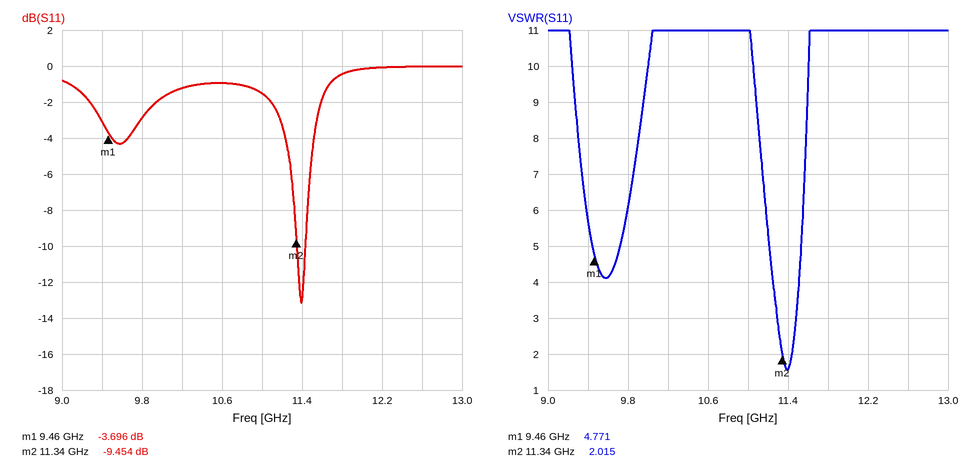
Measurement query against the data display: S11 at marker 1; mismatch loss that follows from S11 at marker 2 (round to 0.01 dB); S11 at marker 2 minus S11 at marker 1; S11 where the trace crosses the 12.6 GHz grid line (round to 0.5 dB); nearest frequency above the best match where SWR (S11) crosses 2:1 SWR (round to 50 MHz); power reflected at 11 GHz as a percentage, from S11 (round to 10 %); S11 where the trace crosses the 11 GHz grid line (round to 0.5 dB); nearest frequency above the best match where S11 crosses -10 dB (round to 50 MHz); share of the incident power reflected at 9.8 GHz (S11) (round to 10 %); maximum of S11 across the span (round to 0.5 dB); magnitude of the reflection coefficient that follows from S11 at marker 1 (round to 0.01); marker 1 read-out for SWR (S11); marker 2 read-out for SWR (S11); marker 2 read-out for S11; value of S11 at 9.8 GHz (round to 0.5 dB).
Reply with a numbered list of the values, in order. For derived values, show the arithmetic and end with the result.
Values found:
1. -3.696 dB
2. −10 log10(1 − 10^(-9.454/10)) ≈ 0.52 dB
3. -9.454 − (-3.696) = -5.758 dB
4. 0.0 dB
5. 11.45 GHz
6. 10^(-1.5/10) ≈ 70.8 %, so 70 % to the nearest 10 %
7. -1.5 dB
8. 11.45 GHz
9. 10^(-3/10) ≈ 50 %
10. 0.0 dB
11. 10^(-3.696/20) ≈ 0.65
12. 4.771
13. 2.015
14. -9.454 dB
15. -3.0 dB
